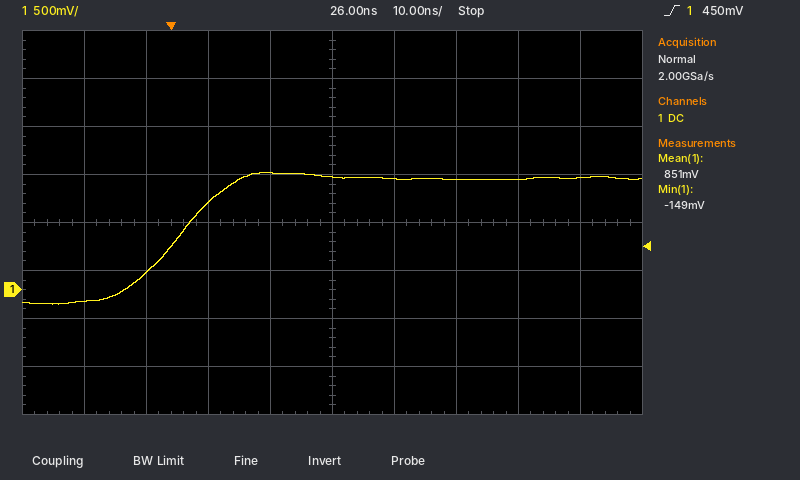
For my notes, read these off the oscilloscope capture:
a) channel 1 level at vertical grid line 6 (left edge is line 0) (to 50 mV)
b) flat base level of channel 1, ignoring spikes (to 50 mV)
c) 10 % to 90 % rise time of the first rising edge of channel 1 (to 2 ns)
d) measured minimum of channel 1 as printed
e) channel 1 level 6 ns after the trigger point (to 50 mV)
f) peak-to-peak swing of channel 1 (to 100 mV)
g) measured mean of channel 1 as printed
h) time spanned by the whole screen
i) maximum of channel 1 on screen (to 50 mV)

1.15 V
-150 mV
16 ns
-149 mV
900 mV
1.40 V
851 mV
100 ns
1.20 V
